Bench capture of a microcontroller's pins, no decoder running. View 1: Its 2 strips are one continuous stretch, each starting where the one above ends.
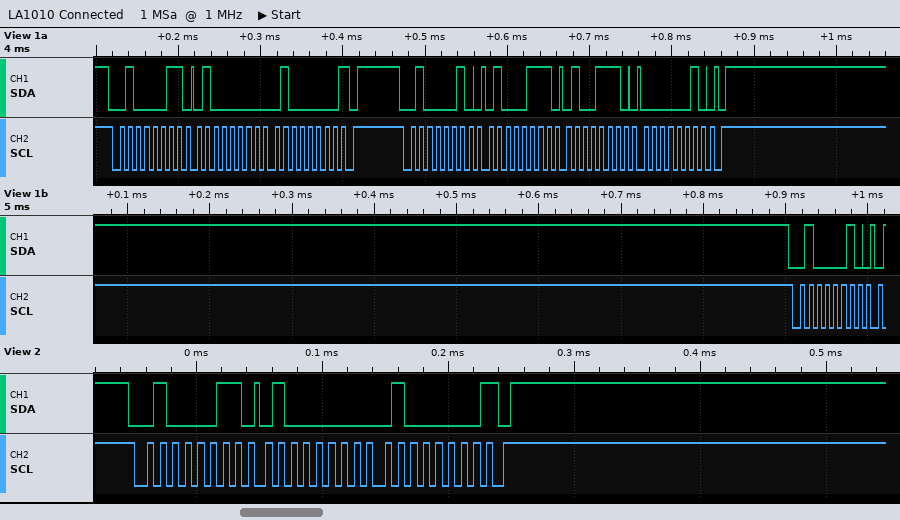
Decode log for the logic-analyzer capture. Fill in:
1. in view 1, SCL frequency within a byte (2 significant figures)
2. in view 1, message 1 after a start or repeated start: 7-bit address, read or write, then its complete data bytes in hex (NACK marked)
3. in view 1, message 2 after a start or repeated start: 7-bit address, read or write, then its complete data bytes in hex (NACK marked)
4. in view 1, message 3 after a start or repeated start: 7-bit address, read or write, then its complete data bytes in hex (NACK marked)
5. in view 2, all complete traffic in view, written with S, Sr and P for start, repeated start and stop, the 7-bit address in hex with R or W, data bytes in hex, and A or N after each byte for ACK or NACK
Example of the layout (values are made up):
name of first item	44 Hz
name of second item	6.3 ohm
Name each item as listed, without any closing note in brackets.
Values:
in view 1, SCL frequency within a byte	100 kHz
in view 1, message 1 after a start or repeated start: 7-bit address, read or write, then its complete data bytes in hex	0x21 read: 40 40 NACK
in view 1, message 2 after a start or repeated start: 7-bit address, read or write, then its complete data bytes in hex	0x21 write: 47 4E 02
in view 1, message 3 after a start or repeated start: 7-bit address, read or write, then its complete data bytes in hex	0x21 write
in view 2, all complete traffic in view, written with S, Sr and P for start, repeated start and stop, the 7-bit address in hex with R or W, data bytes in hex, and A or N after each byte for ACK or NACK	S 21R A 40 A 40 N P
